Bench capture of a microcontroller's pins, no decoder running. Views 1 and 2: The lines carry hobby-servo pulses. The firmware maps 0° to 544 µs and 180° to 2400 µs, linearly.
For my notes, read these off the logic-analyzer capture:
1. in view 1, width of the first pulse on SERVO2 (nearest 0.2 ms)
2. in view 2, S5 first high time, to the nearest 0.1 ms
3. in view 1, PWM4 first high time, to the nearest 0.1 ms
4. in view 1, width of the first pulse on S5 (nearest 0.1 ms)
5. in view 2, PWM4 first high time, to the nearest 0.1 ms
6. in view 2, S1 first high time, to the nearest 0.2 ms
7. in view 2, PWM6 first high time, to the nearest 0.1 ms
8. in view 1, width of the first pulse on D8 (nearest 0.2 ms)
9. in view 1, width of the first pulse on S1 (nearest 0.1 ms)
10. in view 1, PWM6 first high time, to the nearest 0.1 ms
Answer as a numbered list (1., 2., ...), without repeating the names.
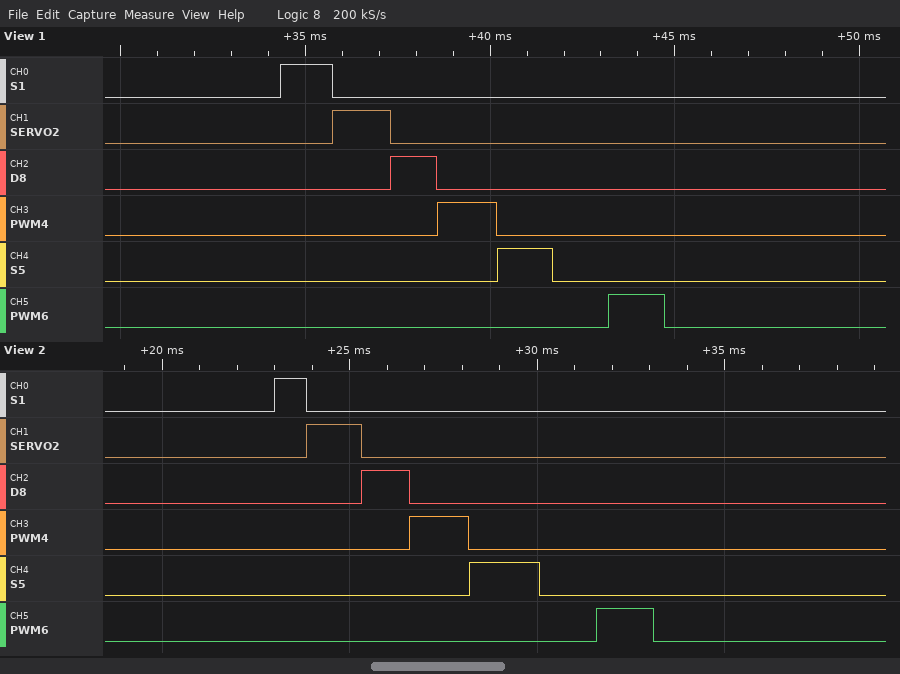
1. 1.6 ms
2. 1.9 ms
3. 1.6 ms
4. 1.5 ms
5. 1.6 ms
6. 0.8 ms
7. 1.5 ms
8. 1.2 ms
9. 1.4 ms
10. 1.5 ms
